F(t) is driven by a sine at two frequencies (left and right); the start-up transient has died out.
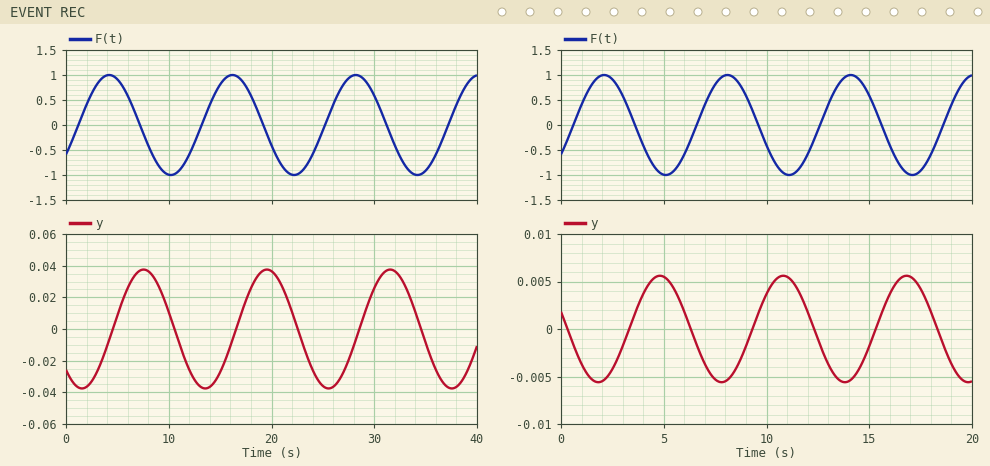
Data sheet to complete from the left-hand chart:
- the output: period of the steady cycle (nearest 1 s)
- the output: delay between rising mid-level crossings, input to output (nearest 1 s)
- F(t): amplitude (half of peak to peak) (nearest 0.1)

12 s
3 s
1.0
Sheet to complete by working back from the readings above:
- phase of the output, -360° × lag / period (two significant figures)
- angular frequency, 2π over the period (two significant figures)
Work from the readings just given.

-90°
0.52 rad/s
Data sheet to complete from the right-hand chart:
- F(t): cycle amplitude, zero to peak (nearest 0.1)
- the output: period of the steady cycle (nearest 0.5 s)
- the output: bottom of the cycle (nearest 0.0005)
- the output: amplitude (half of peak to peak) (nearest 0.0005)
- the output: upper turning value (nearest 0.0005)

1.0
6.0 s
-0.0055
0.0055
0.0055
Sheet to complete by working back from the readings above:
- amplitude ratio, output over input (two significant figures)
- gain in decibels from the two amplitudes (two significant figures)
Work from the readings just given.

0.0055
-45 dB
